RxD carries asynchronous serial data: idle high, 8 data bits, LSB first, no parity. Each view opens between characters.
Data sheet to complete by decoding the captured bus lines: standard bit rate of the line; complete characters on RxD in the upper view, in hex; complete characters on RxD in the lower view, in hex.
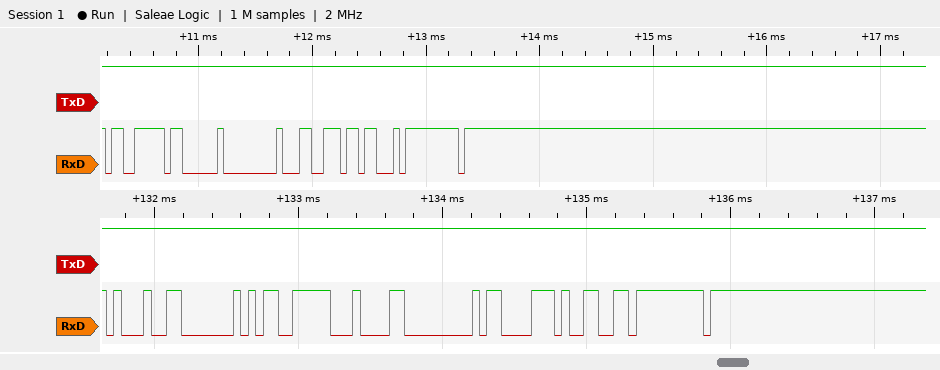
19200 baud
F3, 03, 00, CC, 1B, FF, FF
91, 40, F3, 84, 00, C3, 99, FF, FF
